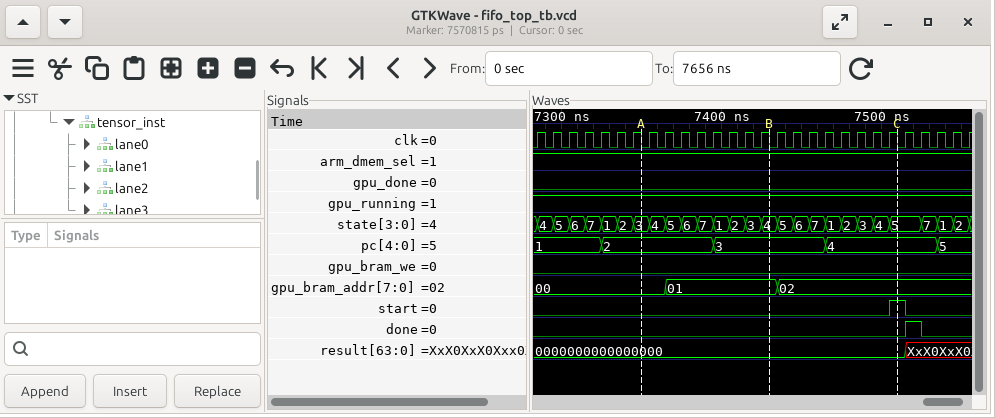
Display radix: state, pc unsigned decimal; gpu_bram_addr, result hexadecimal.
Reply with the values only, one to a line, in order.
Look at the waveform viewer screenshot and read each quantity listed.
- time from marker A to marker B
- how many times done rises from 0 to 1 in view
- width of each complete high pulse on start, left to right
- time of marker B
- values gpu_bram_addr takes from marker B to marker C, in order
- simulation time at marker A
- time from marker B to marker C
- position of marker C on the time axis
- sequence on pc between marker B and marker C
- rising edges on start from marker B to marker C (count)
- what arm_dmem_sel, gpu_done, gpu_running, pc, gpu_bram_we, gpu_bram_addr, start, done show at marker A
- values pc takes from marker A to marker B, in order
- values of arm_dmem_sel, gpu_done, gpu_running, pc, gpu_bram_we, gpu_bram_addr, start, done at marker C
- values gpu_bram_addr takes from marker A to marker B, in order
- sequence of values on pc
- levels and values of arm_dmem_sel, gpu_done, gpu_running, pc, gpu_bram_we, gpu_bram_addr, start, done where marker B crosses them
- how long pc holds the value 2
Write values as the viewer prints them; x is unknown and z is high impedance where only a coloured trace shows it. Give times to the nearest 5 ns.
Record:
80 ns
1
10 ns
7430 ns
01, 02
7350 ns
80 ns
7510 ns
3, 4
1
arm_dmem_sel=1, gpu_done=0, gpu_running=1, pc=2, gpu_bram_we=0, gpu_bram_addr=00, start=0, done=0
2, 3
arm_dmem_sel=1, gpu_done=0, gpu_running=1, pc=4, gpu_bram_we=0, gpu_bram_addr=02, start=1, done=0
00, 01
1, 2, 3, 4, 5
arm_dmem_sel=1, gpu_done=0, gpu_running=1, pc=3, gpu_bram_we=0, gpu_bram_addr=01, start=0, done=0
70 ns
